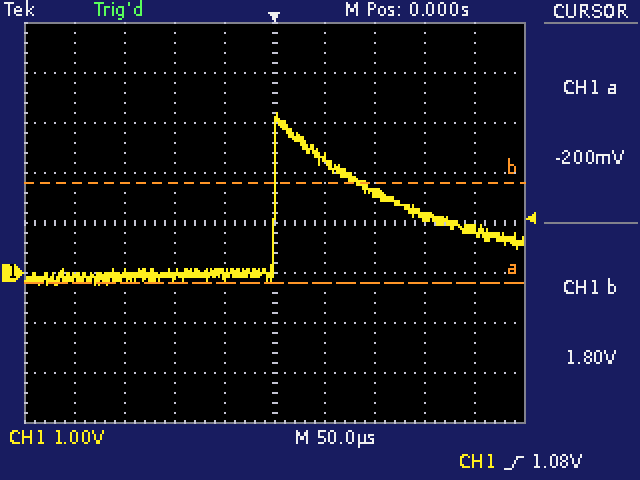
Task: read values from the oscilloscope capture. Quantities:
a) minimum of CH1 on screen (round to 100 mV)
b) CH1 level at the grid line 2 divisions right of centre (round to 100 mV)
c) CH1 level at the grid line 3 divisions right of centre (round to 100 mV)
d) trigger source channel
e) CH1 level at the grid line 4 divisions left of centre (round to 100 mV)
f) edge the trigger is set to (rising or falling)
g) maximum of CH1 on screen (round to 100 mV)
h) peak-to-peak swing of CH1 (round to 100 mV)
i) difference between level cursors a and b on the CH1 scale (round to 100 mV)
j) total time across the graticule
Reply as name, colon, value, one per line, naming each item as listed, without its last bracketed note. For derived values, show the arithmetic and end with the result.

minimum of CH1 on screen: -200 mV
CH1 level at the grid line 2 divisions right of centre: 1.6 V
CH1 level at the grid line 3 divisions right of centre: 1.1 V
trigger source channel: CH1
CH1 level at the grid line 4 divisions left of centre: -100 mV
edge the trigger is set to: rising
maximum of CH1 on screen: 3.2 V
peak-to-peak swing of CH1: 3.2 V − (-200 mV) = 3.4 V
difference between level cursors a and b on the CH1 scale: 2.0 V
total time across the graticule: 500 µs
